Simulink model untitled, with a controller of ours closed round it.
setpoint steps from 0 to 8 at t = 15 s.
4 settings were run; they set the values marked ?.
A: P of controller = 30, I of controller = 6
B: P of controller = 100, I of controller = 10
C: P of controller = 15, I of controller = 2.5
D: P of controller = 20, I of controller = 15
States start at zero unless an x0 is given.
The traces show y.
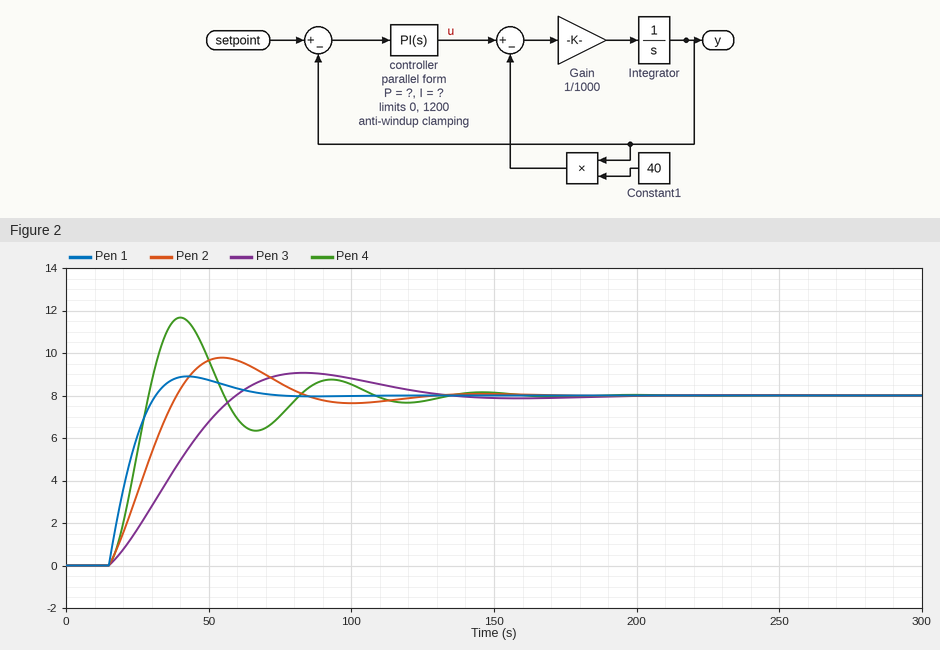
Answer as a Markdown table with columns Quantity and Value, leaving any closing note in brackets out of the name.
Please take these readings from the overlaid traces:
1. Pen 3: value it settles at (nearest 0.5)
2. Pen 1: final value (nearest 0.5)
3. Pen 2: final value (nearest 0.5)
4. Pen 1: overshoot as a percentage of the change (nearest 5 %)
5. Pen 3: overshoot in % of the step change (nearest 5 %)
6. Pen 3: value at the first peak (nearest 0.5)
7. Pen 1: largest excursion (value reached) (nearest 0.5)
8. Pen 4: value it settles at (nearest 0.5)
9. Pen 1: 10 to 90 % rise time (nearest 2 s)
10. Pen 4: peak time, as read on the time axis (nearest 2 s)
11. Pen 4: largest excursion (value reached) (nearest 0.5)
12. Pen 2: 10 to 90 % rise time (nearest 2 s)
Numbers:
| Quantity | Value |
|---|---|
| Pen 3: value it settles at | 8.0 |
| Pen 1: final value | 8.0 |
| Pen 2: final value | 8.0 |
| Pen 1: overshoot as a percentage of the change | 10 % |
| Pen 3: overshoot in % of the step change | 15 % |
| Pen 3: value at the first peak | 9.0 |
| Pen 1: largest excursion (value reached) | 9.0 |
| Pen 4: value it settles at | 8.0 |
| Pen 1: 10 to 90 % rise time | 12 s |
| Pen 4: peak time, as read on the time axis | 40 s |
| Pen 4: largest excursion (value reached) | 11.5 |
| Pen 2: 10 to 90 % rise time | 18 s |
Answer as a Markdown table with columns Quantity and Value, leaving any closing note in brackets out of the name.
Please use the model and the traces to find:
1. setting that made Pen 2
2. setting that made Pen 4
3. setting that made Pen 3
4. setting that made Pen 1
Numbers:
| Quantity | Value |
|---|---|
| setting that made Pen 2 | A |
| setting that made Pen 4 | D |
| setting that made Pen 3 | C |
| setting that made Pen 1 | B |
